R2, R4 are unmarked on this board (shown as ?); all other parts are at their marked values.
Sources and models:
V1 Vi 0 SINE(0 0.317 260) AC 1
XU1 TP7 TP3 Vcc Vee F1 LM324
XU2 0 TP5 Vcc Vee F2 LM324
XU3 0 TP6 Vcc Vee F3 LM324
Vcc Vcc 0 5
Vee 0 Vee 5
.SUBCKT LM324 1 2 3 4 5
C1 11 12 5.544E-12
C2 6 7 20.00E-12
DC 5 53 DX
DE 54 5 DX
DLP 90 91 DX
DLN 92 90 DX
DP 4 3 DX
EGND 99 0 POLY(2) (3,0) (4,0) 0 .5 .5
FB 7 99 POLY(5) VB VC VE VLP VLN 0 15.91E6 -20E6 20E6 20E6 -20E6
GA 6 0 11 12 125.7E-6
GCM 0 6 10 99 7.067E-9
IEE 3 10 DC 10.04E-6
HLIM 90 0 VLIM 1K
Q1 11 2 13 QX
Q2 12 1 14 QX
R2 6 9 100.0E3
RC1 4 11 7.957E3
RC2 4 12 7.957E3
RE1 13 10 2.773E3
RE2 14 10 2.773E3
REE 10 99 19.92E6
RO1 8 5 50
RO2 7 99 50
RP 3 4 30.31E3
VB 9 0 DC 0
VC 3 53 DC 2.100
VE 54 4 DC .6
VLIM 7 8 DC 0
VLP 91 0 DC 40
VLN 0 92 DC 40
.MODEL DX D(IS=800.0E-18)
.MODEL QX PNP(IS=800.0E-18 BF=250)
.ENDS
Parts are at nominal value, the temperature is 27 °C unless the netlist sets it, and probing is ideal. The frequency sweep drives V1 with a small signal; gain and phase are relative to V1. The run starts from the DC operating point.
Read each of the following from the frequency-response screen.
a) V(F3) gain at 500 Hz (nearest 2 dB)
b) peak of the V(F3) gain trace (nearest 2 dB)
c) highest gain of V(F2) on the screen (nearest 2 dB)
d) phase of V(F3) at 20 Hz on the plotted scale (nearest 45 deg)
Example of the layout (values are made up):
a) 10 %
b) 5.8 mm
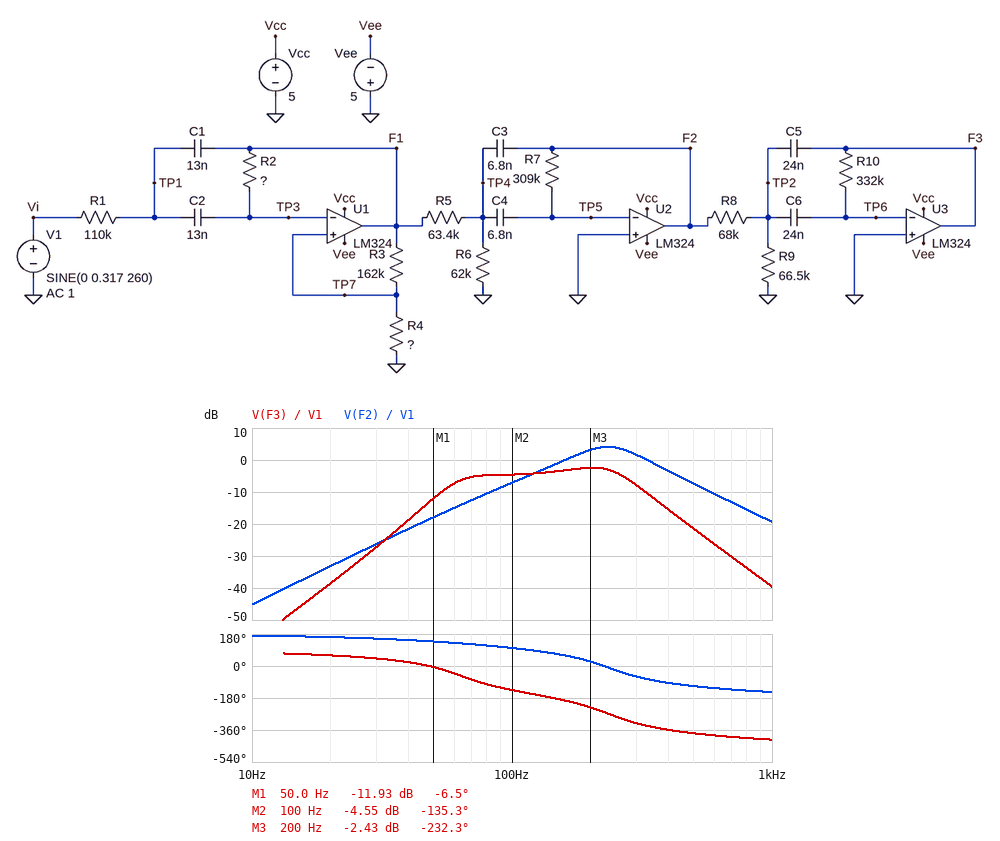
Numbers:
a) -22 dB
b) -2 dB
c) 4 dB
d) 45 deg
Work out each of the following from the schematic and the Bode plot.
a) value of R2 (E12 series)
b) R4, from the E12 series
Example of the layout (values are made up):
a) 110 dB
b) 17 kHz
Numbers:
a) 39 kΩ
b) 270 kΩ
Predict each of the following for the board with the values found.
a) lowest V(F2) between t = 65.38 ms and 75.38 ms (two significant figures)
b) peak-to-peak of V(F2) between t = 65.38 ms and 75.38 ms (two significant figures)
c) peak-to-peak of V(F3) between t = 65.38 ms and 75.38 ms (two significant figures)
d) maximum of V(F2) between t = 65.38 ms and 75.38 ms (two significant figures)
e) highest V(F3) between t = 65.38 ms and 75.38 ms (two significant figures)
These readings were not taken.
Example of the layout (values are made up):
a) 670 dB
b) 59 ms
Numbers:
a) -490 mV
b) 960 mV
c) 380 mV
d) 470 mV
e) 180 mV
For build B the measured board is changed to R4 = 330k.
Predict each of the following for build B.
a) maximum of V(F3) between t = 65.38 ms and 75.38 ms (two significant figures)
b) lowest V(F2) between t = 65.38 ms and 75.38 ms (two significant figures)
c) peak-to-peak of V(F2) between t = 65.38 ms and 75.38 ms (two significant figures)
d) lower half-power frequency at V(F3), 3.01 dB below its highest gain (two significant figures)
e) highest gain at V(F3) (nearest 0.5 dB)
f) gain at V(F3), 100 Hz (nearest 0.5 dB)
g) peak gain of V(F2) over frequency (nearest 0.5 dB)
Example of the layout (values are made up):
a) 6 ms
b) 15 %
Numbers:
a) 230 mV
b) -600 mV
c) 1.2 V
d) 73 Hz
e) -0.5 dB
f) -3.0 dB
g) 6.0 dB
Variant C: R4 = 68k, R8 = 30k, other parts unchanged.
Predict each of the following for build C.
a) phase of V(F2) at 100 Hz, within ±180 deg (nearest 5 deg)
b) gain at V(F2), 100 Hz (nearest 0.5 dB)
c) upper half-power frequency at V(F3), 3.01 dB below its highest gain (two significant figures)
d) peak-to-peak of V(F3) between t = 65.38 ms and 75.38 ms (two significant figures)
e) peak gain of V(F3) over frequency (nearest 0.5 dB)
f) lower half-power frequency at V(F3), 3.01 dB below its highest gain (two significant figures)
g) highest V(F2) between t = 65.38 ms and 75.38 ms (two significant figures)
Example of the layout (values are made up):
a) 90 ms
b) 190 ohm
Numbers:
a) 95 deg
b) -14.5 dB
c) 260 Hz
d) 370 mV
e) -2.0 dB
f) 72 Hz
g) 190 mV
